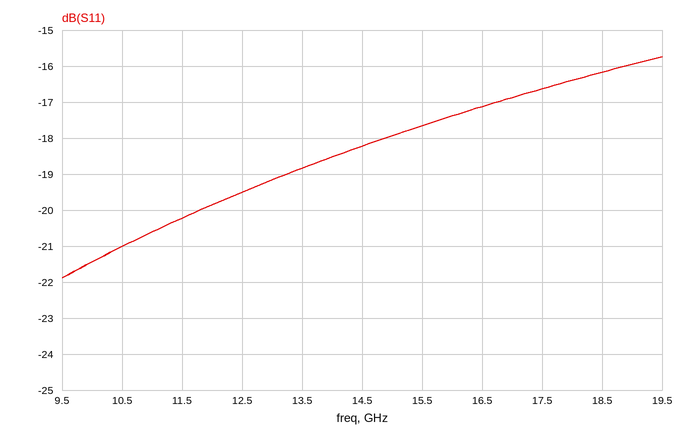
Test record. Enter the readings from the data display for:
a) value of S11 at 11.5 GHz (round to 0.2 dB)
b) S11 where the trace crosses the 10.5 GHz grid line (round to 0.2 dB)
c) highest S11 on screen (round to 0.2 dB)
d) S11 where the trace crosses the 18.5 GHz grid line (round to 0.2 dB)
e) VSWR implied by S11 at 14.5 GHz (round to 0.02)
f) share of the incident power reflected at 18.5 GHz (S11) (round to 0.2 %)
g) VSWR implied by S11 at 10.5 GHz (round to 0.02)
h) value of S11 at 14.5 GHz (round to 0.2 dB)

-20.2 dB
-21.0 dB
-15.8 dB
-16.2 dB
1.28
2.4 %
1.20
-18.2 dB
